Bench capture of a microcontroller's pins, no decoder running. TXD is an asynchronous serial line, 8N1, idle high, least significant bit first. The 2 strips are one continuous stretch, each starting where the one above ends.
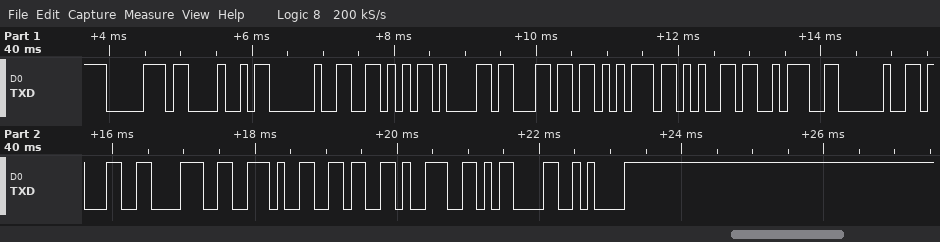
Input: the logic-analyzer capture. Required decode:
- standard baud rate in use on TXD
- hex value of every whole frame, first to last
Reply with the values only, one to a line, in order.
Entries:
9600 baud
0x70 0x48 0x20 0x56 0x61 0x6C 0x75 0x65 0x3A 0x20 0x31 0x38 0x2E 0x36 0x39 0x0D 0x0A
